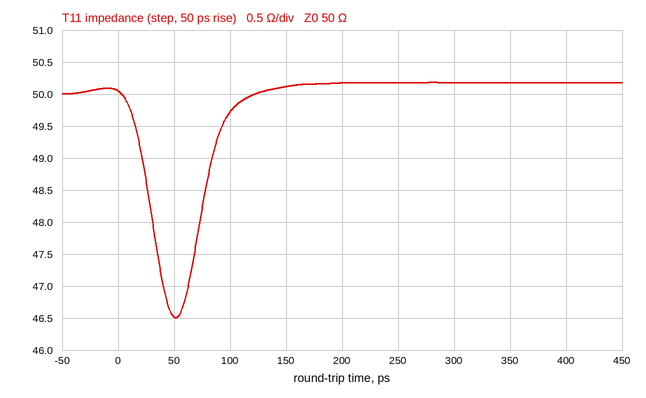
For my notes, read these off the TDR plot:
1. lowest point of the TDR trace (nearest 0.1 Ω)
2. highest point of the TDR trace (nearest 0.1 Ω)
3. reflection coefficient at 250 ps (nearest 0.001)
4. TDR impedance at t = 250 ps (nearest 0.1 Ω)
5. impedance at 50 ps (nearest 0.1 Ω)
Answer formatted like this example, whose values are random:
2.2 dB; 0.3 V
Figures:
46.5 Ω; 50.2 Ω; +0.002; 50.2 Ω; 46.5 Ω
